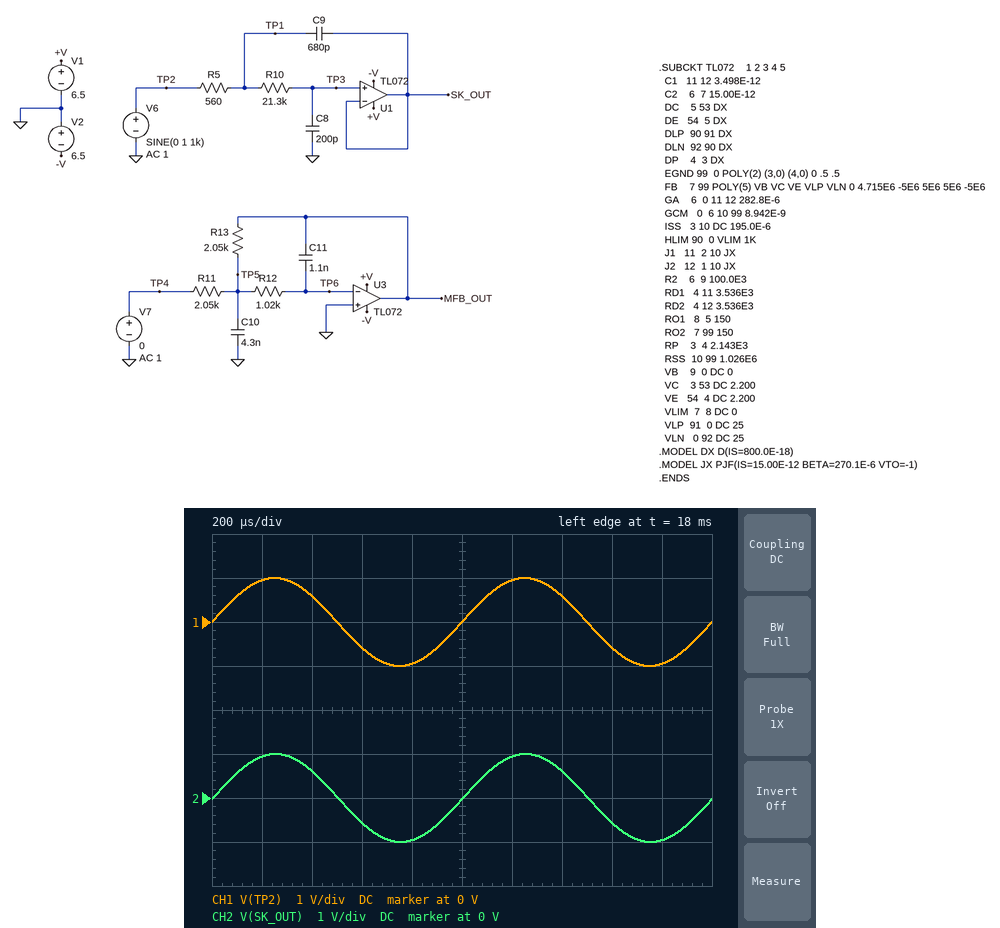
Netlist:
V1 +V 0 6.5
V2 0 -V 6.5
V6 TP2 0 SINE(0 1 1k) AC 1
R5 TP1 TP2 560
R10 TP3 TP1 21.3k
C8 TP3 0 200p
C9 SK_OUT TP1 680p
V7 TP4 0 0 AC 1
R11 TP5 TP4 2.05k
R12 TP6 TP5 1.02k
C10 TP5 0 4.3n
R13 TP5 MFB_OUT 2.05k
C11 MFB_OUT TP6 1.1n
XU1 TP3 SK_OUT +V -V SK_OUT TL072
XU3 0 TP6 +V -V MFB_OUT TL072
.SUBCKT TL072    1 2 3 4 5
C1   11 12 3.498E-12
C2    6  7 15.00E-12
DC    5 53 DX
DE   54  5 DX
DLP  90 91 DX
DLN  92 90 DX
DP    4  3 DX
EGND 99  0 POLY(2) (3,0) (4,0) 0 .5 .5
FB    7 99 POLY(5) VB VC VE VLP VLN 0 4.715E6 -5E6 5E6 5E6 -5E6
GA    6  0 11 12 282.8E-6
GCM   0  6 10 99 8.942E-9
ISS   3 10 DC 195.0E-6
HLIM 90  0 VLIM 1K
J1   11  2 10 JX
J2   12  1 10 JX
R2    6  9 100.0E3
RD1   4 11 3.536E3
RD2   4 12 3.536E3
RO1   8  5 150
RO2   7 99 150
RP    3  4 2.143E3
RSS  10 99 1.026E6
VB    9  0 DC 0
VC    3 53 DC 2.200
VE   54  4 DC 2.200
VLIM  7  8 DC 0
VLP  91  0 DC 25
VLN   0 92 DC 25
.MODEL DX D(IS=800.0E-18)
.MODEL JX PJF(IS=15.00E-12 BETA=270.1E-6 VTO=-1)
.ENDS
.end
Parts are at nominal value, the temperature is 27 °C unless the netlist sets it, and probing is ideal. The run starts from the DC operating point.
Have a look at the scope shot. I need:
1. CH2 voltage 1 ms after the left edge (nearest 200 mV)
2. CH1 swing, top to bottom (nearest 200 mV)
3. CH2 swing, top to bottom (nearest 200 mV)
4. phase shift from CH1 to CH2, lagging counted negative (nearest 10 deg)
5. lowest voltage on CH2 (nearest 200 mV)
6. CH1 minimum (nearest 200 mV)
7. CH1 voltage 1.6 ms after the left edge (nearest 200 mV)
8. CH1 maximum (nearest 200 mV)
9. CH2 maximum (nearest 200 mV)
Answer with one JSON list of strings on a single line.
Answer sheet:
["0 V", "2.0 V", "2.0 V", "0 deg", "-1.0 V", "-1.0 V", "-600 mV", "1.0 V", "1.0 V"]
